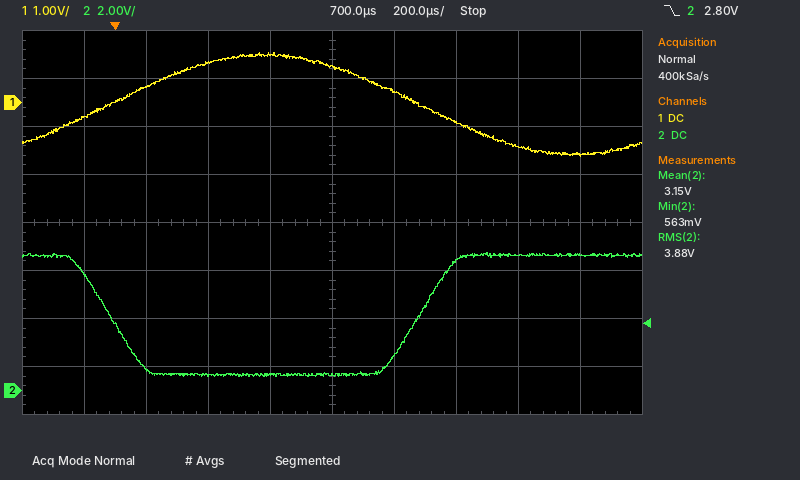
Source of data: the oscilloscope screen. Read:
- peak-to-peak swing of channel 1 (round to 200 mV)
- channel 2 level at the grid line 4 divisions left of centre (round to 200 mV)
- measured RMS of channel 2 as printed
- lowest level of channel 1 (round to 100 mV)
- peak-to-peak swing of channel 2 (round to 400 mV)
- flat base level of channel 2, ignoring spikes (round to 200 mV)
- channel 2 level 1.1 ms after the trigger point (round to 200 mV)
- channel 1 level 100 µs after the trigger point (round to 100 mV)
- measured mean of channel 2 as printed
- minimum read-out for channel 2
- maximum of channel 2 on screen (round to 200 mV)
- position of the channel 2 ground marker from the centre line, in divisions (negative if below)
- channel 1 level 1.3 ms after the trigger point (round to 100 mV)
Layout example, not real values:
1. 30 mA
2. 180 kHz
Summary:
1. 2.2 V
2. 4.8 V
3. 3.88 V
4. -1.1 V
5. 5.2 V
6. 600 mV
7. 5.4 V
8. 300 mV
9. 3.15 V
10. 563 mV
11. 5.8 V
12. -3.5 div
13. -900 mV
